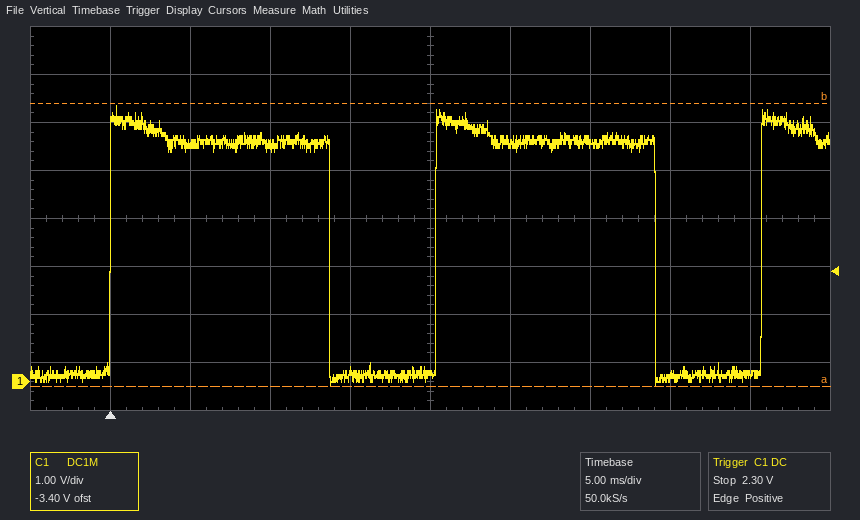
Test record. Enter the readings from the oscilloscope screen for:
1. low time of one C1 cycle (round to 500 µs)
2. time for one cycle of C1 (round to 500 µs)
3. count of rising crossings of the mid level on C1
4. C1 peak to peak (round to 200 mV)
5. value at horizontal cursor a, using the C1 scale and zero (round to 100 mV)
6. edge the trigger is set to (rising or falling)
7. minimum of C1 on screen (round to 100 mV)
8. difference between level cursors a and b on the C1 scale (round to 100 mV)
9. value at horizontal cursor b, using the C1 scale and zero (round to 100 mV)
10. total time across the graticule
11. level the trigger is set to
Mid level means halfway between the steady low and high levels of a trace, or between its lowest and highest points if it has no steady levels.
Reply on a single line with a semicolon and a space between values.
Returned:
6.5 ms; 20.5 ms; 3; 5.8 V; -100 mV; rising; -100 mV; 5.9 V; 5.8 V; 50 ms; 2.30 V
